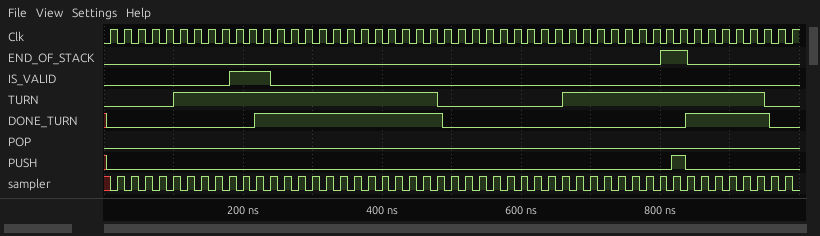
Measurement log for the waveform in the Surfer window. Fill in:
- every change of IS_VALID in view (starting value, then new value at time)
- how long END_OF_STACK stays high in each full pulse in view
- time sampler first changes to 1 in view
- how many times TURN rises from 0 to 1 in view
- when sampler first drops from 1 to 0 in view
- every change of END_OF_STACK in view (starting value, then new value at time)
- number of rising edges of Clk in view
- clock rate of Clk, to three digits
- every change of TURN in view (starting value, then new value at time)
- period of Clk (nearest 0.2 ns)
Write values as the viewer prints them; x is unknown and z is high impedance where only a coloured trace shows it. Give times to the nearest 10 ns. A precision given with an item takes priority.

0, 1 at 180 ns, 0 at 240 ns
40 ns
20 ns
2
30 ns
0, 1 at 800 ns, 0 at 840 ns
50
50.0 MHz
0, 1 at 100 ns, 0 at 480 ns, 1 at 660 ns, 0 at 950 ns
20 ns
